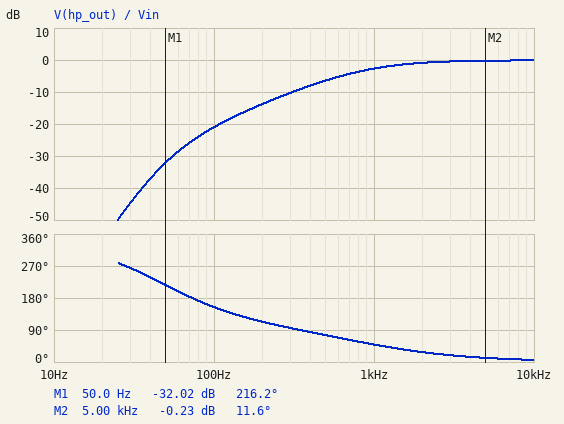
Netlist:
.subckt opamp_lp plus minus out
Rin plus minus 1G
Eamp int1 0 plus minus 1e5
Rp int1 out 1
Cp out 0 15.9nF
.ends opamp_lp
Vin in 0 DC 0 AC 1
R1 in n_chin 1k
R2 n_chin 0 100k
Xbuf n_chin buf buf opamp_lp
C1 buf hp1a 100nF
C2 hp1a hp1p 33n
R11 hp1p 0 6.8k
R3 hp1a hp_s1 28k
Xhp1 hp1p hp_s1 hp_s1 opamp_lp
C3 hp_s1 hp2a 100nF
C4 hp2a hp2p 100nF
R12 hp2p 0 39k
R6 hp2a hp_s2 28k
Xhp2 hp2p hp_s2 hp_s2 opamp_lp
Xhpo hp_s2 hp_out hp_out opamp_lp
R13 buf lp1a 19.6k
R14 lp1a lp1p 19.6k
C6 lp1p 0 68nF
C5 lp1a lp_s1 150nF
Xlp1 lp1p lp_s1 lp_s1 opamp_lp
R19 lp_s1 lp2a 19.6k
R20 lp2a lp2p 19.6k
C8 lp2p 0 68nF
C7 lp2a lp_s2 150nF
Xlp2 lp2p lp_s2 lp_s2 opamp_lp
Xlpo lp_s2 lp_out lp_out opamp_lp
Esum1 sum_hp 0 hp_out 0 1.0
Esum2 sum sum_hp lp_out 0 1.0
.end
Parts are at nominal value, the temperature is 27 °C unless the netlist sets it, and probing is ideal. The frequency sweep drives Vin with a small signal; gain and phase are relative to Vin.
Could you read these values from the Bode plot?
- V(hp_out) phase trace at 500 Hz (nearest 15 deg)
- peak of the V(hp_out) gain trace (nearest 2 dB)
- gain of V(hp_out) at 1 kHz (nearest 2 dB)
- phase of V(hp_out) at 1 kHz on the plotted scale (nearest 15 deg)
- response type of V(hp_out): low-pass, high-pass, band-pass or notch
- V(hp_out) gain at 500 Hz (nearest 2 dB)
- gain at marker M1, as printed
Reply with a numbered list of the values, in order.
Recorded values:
1. 75 deg
2. 0 dB
3. -2 dB
4. 45 deg
5. high-pass
6. -6 dB
7. -32.02 dB
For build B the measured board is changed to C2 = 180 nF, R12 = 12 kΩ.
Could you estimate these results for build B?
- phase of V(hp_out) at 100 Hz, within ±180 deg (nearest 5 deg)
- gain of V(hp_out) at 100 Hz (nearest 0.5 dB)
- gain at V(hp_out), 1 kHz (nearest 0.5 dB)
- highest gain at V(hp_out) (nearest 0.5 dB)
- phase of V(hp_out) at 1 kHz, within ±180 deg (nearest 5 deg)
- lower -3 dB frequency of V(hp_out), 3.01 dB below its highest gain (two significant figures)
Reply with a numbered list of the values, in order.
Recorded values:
1. 170 deg
2. -20.0 dB
3. -1.0 dB
4. 0 dB
5. 35 deg
6. 450 Hz
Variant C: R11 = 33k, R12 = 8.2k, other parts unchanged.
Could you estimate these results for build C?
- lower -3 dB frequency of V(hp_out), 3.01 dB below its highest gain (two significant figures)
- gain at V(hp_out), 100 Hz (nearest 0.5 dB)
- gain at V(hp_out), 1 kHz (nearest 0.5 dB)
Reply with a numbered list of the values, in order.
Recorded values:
1. 410 Hz
2. -17.5 dB
3. -0.5 dB
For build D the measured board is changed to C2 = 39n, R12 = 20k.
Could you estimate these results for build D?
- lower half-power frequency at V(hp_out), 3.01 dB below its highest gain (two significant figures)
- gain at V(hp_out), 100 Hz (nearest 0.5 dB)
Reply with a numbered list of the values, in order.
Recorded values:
1. 810 Hz
2. -23.5 dB
